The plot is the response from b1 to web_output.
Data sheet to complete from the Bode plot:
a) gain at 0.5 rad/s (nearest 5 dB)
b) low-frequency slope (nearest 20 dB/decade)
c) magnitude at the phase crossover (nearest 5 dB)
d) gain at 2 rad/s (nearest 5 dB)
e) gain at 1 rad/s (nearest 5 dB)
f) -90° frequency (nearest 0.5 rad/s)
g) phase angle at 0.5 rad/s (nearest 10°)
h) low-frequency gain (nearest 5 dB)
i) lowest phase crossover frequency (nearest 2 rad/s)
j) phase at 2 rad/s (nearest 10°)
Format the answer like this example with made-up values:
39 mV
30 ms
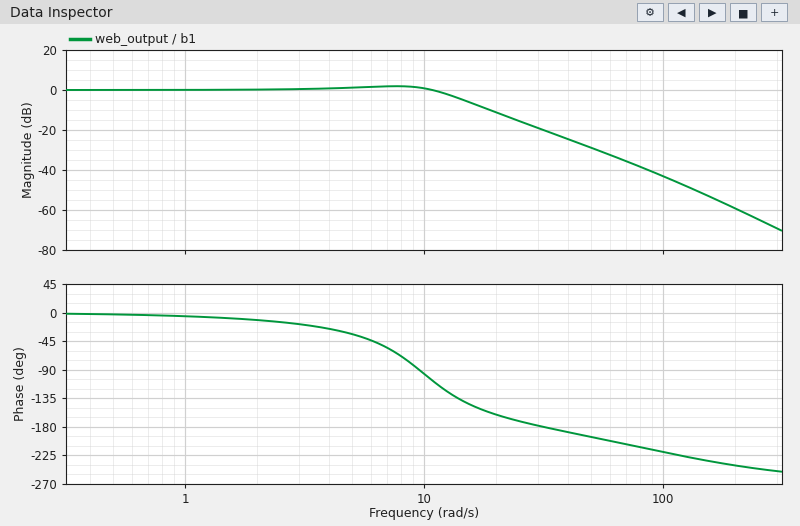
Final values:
0 dB
0 dB/decade
-20 dB
0 dB
0 dB
9.5 rad/s
0°
0 dB
32 rad/s
-10°
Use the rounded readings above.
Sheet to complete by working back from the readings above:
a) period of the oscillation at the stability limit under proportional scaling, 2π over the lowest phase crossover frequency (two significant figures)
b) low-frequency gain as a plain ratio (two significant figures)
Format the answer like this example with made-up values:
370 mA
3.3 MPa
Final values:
0.20 s
1.0
